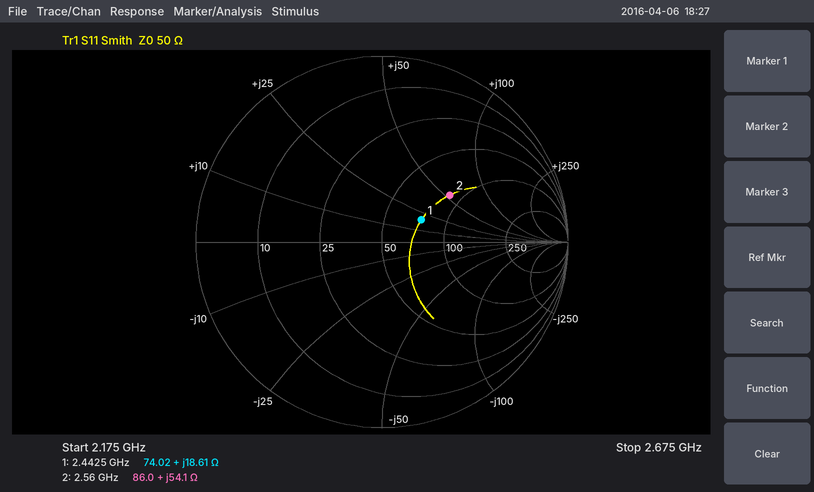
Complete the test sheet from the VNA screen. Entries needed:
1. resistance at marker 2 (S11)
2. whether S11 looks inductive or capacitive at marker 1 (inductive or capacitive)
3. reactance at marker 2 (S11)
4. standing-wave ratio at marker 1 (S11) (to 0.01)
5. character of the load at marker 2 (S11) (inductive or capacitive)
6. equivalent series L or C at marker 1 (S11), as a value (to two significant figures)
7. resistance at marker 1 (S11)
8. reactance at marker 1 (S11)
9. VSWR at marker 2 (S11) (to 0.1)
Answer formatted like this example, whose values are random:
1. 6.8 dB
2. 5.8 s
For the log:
1. 86.0 Ω
2. inductive
3. +54.1 Ω
4. 1.64
5. inductive
6. 1.2 nH
7. 74.02 Ω
8. +18.61 Ω
9. 2.6
